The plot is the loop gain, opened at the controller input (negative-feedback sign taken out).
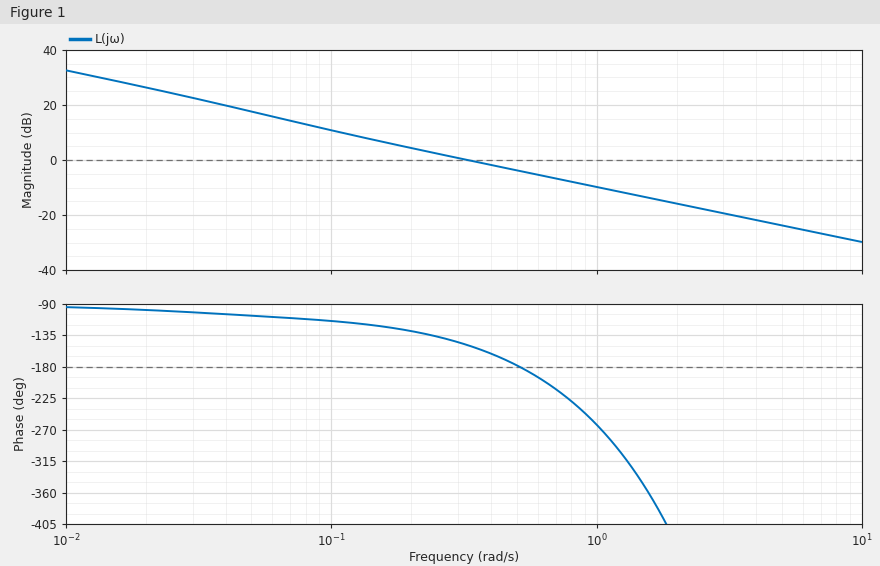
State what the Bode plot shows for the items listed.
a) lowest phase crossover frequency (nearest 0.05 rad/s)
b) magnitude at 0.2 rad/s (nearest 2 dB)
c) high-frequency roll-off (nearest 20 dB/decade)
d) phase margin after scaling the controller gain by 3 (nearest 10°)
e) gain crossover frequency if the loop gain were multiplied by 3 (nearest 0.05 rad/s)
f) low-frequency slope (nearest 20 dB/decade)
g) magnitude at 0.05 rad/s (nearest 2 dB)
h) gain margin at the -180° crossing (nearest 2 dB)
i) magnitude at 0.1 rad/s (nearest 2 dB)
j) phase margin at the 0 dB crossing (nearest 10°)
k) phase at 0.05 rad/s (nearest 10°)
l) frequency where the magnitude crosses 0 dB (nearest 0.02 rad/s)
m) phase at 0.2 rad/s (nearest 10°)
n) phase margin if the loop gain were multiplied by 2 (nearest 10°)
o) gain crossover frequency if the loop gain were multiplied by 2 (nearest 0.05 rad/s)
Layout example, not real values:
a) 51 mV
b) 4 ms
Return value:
a) 0.50 rad/s
b) 4 dB
c) -20 dB/decade
d) -80°
e) 0.95 rad/s
f) -20 dB/decade
g) 18 dB
h) 4 dB
i) 10 dB
j) 30°
k) -110°
l) 0.32 rad/s
m) -130°
n) -20°
o) 0.65 rad/s
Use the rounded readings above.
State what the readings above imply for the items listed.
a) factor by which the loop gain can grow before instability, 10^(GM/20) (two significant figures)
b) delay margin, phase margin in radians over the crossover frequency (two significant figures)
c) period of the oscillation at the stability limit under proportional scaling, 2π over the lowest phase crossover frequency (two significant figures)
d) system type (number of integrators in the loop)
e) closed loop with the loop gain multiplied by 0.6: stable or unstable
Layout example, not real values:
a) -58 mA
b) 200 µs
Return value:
a) 1.6
b) 1.6 s
c) 13 s
d) 1
e) stable
